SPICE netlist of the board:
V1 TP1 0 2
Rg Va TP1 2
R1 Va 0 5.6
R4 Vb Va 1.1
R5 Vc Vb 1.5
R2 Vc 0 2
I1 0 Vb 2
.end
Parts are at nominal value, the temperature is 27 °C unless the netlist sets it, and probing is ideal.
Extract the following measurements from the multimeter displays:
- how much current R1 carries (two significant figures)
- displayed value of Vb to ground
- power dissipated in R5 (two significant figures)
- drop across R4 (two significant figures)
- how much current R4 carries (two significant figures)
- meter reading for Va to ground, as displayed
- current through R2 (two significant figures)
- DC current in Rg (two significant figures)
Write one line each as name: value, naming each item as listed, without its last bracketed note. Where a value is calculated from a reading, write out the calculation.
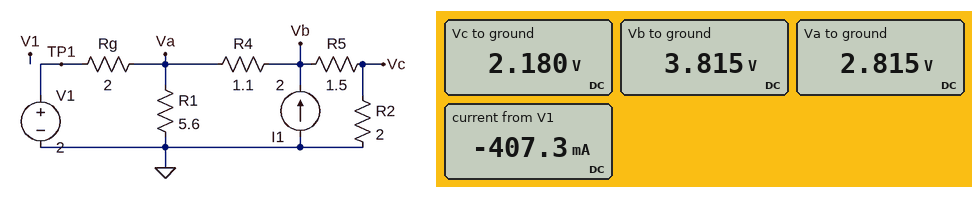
how much current R1 carries: (2.815 V) / 5.6 Ω = 500 mA
displayed value of Vb to ground: 3.815 V
power dissipated in R5: (3.815 V - 2.18 V)^2 / 1.5 Ω = 1.8 W
drop across R4: 3.815 V - 2.815 V = 1.0 V
how much current R4 carries: (3.815 V - 2.815 V) / 1.1 Ω = 910 mA
meter reading for Va to ground, as displayed: 2.815 V
current through R2: (2.18 V) / 2 Ω = 1.1 A
DC current in Rg: (2.815 V - 2 V) / 2 Ω = 410 mA
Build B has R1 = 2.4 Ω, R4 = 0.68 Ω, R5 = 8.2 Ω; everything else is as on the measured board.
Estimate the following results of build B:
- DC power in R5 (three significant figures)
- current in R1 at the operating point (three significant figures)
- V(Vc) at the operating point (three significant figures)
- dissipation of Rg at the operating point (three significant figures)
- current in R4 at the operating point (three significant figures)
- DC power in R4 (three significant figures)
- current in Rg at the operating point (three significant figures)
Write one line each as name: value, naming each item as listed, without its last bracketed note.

DC power in R5: 1.23 W
current in R1 at the operating point: 1.19 A
V(Vc) at the operating point: 774 mV
dissipation of Rg at the operating point: 362 mW
current in R4 at the operating point: 1.61 A
DC power in R4: 1.77 W
current in Rg at the operating point: 425 mA
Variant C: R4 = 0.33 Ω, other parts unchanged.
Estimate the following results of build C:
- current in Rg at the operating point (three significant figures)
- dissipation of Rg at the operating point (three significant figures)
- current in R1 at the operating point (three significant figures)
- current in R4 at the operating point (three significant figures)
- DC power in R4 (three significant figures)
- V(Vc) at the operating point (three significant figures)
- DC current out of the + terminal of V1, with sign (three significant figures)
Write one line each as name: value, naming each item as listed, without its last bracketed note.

current in Rg at the operating point: 505 mA
dissipation of Rg at the operating point: 509 mW
current in R1 at the operating point: 537 mA
current in R4 at the operating point: 1.04 A
DC power in R4: 358 mW
V(Vc) at the operating point: 1.92 V
DC current out of the + terminal of V1, with sign: -505 mA
